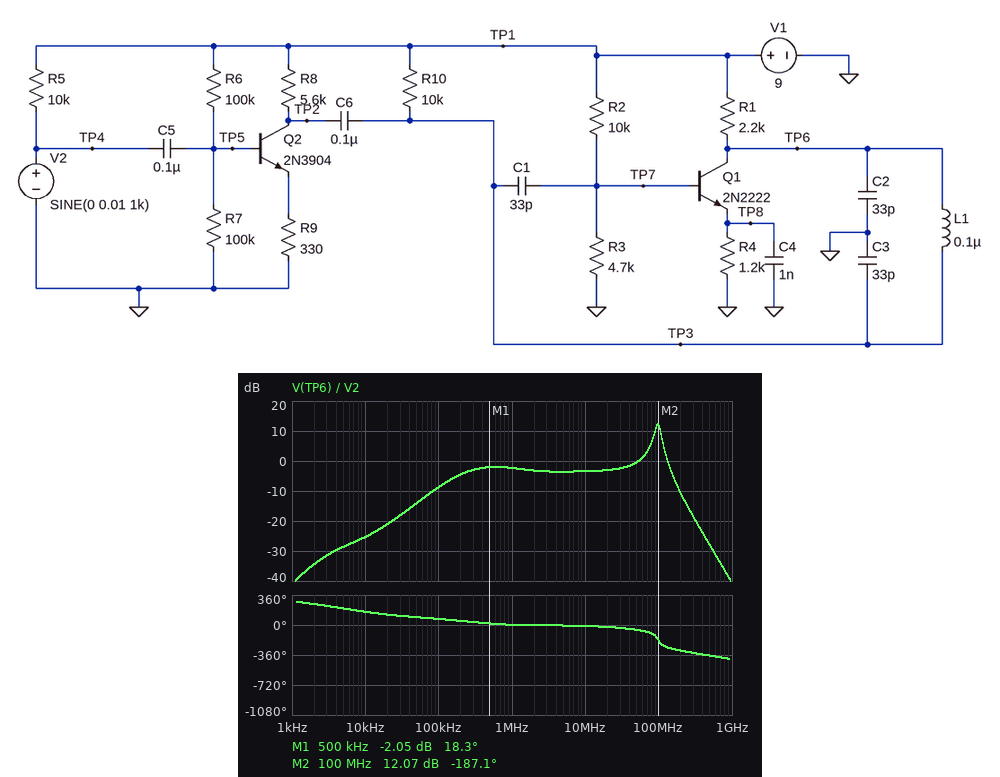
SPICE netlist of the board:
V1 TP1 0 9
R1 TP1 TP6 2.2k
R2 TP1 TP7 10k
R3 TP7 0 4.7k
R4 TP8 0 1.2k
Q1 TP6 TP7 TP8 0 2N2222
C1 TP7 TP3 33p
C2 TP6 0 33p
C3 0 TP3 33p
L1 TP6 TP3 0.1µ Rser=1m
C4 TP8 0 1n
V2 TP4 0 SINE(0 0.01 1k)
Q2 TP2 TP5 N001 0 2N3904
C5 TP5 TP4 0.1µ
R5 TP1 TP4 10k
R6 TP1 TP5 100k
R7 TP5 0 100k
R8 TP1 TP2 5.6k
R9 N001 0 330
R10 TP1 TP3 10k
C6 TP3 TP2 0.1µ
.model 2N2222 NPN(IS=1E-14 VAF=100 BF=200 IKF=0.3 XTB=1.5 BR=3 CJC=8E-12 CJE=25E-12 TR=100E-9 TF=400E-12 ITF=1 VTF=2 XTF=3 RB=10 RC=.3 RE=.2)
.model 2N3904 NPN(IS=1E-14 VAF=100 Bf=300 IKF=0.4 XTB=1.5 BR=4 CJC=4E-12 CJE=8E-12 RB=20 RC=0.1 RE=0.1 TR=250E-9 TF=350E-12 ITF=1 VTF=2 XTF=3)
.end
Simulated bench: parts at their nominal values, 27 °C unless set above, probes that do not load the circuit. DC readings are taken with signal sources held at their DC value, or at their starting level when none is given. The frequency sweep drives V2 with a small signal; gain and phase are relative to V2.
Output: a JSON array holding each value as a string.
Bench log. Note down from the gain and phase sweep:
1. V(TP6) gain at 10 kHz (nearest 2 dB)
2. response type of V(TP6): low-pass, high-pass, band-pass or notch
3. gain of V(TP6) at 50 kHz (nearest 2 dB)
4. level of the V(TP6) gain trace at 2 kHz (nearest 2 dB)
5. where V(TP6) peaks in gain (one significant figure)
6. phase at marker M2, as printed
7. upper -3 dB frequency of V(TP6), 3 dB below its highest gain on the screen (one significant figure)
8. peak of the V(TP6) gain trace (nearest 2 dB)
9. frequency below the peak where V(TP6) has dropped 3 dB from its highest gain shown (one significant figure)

["-26 dB", "band-pass", "-14 dB", "-34 dB", "100 MHz", "-187.1 deg", "100 MHz", "12 dB", "90 MHz"]
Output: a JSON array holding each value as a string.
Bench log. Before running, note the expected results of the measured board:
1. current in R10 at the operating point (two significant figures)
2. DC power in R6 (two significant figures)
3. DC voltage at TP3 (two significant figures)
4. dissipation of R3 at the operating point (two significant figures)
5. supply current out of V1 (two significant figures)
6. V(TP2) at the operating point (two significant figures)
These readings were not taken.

["330 µA", "610 µW", "5.7 V", "1.7 mW", "4.9 mA", "570 mV"]
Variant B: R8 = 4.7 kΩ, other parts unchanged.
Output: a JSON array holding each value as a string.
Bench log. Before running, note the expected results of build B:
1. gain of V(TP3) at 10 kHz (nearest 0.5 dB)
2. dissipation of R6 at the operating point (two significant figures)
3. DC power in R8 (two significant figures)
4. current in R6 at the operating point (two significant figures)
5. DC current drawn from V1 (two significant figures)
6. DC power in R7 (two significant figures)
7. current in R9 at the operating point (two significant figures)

["-20.5 dB", "600 µW", "15 mW", "77 µA", "5.2 mA", "16 µW", "1.8 mA"]
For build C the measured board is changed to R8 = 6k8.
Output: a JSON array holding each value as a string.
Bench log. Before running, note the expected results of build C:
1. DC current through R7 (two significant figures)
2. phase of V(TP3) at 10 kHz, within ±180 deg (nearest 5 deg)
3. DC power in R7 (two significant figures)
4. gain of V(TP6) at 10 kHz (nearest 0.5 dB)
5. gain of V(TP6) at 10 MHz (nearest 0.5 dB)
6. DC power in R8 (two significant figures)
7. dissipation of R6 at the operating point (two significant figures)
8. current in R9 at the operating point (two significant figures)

["11 µA", "100 deg", "12 µW", "-28.5 dB", "-3.5 dB", "11 mW", "620 µW", "1.3 mA"]
